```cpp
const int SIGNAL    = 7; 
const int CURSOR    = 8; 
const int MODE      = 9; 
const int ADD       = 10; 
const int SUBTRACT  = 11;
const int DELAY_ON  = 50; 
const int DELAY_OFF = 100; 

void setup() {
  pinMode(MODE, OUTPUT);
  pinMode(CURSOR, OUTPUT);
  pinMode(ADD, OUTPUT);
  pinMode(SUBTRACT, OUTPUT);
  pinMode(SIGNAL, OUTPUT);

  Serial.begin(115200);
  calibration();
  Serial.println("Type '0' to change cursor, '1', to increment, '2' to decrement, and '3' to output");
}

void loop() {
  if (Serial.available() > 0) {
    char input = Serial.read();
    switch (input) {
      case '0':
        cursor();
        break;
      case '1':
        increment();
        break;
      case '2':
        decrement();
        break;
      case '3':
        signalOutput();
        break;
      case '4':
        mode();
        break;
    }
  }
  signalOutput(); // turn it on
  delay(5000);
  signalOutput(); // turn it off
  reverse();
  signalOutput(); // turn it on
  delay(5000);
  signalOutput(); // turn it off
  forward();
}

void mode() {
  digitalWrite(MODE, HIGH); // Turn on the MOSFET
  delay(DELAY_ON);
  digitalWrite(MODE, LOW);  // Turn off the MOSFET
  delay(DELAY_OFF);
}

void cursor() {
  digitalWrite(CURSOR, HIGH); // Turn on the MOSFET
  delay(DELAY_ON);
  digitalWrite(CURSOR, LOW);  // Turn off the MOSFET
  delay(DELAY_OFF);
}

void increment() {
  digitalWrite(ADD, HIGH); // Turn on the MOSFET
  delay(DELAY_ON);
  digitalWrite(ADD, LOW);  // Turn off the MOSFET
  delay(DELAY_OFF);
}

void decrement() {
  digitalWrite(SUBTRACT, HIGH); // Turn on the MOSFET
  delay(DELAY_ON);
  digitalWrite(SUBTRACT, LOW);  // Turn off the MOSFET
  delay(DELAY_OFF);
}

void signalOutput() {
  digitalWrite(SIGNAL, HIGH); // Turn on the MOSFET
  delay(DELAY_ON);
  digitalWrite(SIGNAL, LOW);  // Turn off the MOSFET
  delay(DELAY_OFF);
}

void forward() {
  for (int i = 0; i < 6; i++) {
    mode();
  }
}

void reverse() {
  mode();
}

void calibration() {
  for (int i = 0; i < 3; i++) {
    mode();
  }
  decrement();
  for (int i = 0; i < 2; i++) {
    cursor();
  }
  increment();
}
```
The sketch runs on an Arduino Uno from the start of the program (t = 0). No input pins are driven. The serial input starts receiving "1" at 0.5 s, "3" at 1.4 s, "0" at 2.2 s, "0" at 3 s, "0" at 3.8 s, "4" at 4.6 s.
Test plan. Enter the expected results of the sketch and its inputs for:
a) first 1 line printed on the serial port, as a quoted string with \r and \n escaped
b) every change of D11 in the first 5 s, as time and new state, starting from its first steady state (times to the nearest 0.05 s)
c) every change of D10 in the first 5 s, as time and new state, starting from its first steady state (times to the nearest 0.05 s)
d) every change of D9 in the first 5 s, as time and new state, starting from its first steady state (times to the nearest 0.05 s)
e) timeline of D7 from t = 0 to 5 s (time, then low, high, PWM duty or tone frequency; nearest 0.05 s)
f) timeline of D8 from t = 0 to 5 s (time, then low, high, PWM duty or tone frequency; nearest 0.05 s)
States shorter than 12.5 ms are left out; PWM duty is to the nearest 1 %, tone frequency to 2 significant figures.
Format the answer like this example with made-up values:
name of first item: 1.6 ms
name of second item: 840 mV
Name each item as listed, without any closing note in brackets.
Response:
first 1 line printed on the serial port, as a quoted string with \r and \n escaped: "Type '0' to change cursor, '1', to increment, '2' to decrement, and '3' to output\r\n"
every change of D11 in the first 5 s, as time and new state, starting from its first steady state: 0 s low; 0.45 s high; 0.5 s low
every change of D10 in the first 5 s, as time and new state, starting from its first steady state: 0 s low; 0.9 s high; 0.95 s low; 1.05 s high; 1.1 s low
every change of D9 in the first 5 s, as time and new state, starting from its first steady state: 0 s high; 0.05 s low; 0.15 s high; 0.2 s low; 0.3 s high; 0.35 s low
timeline of D7 from t = 0 to 5 s: 0 s low; 1.2 s high; 1.25 s low
timeline of D8 from t = 0 to 5 s: 0 s low; 0.6 s high; 0.65 s low; 0.75 s high; 0.8 s low
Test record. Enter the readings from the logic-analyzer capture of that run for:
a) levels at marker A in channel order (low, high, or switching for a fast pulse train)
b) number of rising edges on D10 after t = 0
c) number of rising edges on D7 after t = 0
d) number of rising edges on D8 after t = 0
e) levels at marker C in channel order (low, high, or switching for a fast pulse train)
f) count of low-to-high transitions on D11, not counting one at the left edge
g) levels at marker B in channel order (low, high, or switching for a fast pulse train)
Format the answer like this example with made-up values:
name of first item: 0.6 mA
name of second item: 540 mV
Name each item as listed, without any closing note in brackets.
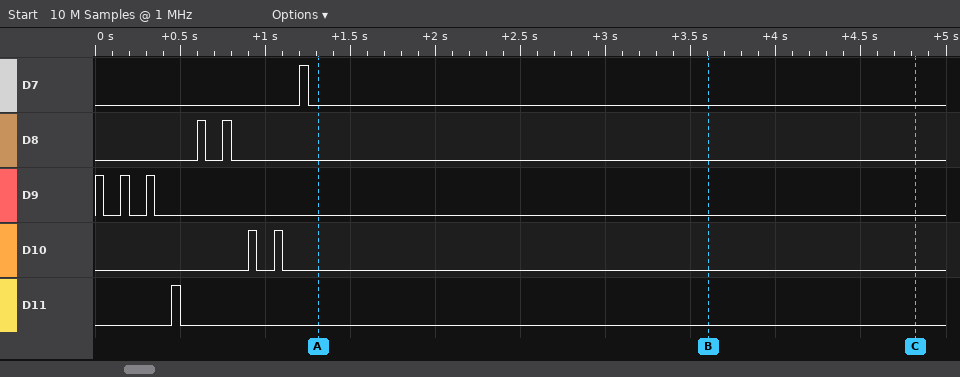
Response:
levels at marker A in channel order: D7 low, D8 low, D9 low, D10 low, D11 low
number of rising edges on D10 after t = 0: 2
number of rising edges on D7 after t = 0: 1
number of rising edges on D8 after t = 0: 2
levels at marker C in channel order: D7 low, D8 low, D9 low, D10 low, D11 low
count of low-to-high transitions on D11, not counting one at the left edge: 1
levels at marker B in channel order: D7 low, D8 low, D9 low, D10 low, D11 low
